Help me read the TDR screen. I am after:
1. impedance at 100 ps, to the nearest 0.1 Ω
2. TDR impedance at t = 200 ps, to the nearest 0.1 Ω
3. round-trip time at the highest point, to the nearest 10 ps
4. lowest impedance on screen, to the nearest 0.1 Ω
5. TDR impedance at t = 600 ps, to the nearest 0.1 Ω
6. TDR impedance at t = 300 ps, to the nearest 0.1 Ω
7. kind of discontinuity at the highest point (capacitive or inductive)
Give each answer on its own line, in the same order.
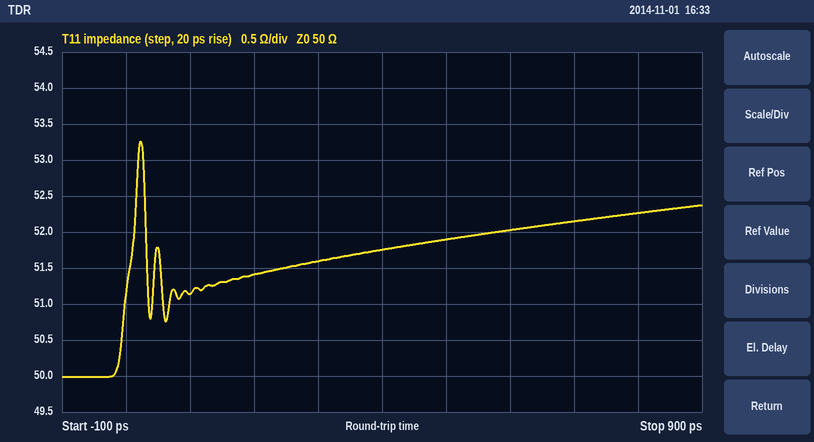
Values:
51.1 Ω
51.4 Ω
20 ps
50.0 Ω
52.0 Ω
51.6 Ω
inductive
